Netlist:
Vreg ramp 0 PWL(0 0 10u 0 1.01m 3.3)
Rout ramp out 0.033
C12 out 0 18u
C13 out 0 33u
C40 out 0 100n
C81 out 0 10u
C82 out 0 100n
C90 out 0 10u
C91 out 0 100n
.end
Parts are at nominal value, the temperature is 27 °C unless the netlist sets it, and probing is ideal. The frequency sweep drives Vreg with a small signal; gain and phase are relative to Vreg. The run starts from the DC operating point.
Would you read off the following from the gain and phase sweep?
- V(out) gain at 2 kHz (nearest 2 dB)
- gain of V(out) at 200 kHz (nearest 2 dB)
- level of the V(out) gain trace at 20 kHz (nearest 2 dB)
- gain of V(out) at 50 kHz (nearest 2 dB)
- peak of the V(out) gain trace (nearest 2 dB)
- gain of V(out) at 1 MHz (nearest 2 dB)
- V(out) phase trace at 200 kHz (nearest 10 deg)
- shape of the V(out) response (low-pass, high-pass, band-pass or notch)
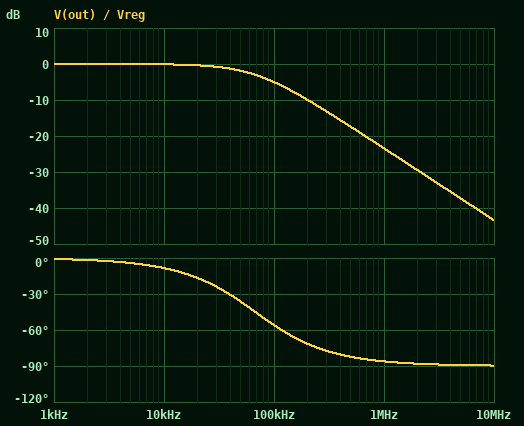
0 dB
-10 dB
0 dB
-2 dB
0 dB
-24 dB
-70 deg
low-pass
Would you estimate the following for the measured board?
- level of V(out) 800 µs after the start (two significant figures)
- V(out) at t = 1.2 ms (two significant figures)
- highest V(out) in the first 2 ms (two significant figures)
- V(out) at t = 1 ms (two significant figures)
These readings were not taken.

2.6 V
3.3 V
3.3 V
3.3 V
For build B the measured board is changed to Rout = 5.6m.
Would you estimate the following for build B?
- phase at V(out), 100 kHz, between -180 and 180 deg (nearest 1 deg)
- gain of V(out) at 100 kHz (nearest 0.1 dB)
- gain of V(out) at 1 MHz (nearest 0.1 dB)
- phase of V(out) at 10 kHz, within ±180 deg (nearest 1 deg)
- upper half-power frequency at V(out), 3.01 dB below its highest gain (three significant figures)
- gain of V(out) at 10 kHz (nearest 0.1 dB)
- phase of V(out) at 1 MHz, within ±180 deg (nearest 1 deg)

-14 deg
-0.3 dB
-8.6 dB
-1 deg
399 kHz
0 dB
-68 deg
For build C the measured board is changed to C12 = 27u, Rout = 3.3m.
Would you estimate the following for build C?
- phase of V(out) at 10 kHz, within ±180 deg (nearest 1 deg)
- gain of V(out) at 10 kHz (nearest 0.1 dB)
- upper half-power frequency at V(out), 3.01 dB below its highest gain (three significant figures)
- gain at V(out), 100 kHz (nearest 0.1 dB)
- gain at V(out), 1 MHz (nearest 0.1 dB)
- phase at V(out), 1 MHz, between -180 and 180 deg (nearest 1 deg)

-1 deg
0 dB
601 kHz
-0.1 dB
-5.8 dB
-59 deg
